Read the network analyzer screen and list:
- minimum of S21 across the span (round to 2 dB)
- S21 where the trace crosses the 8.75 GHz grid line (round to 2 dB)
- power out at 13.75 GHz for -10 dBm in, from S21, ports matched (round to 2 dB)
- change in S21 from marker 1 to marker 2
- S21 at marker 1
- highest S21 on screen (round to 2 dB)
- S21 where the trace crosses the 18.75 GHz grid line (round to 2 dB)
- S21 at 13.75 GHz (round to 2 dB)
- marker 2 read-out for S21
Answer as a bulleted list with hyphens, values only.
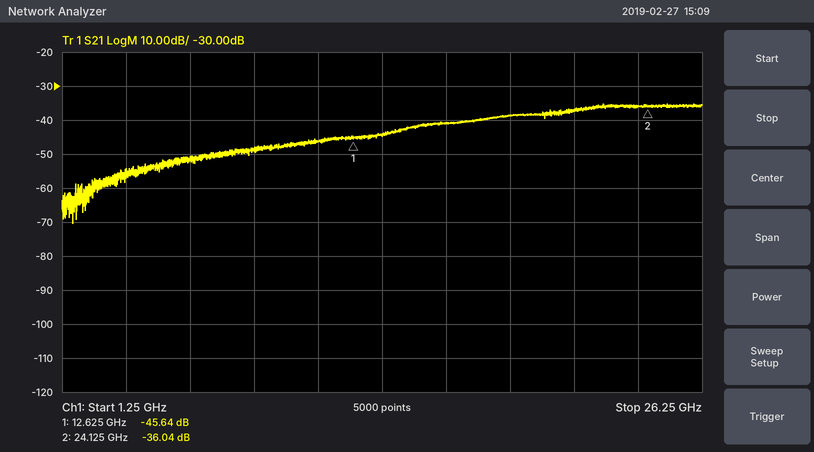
- -70 dB
- -48 dB
- -54 dBm
- 9.60 dB
- -45.64 dB
- -36 dB
- -38 dB
- -44 dB
- -36.04 dB
